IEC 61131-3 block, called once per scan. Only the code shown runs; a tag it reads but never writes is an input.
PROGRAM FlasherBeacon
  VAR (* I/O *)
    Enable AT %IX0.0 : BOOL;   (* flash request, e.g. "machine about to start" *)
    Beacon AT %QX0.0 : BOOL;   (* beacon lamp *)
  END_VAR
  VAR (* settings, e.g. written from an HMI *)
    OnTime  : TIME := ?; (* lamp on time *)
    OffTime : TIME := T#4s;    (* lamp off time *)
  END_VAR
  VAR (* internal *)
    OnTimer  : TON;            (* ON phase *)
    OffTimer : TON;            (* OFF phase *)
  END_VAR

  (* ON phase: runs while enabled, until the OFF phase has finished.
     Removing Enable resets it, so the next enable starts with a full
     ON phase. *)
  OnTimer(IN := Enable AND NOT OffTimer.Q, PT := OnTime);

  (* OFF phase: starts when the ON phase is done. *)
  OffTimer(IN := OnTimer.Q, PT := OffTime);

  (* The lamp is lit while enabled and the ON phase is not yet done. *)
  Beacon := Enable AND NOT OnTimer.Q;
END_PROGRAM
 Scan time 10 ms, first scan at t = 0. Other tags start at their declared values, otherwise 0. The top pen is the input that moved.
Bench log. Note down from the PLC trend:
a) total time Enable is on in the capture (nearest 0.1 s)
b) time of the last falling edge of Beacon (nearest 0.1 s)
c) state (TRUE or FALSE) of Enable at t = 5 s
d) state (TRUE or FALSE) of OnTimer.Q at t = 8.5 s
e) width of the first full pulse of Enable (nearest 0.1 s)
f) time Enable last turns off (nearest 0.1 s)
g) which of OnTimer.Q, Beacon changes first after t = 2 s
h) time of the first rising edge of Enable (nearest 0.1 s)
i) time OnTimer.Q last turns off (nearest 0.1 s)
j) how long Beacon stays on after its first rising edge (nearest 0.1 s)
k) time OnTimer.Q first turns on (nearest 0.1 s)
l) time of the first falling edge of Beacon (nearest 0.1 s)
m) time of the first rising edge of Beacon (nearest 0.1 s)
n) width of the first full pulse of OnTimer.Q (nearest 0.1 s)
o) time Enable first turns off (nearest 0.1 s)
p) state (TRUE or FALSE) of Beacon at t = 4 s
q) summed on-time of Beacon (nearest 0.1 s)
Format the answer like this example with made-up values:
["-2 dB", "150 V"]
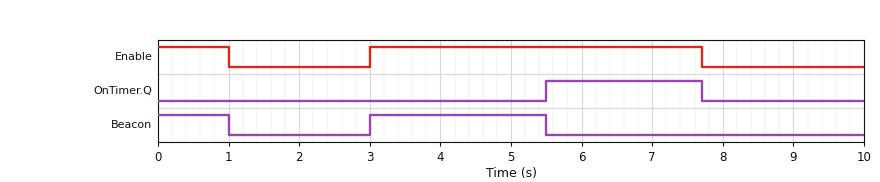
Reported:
["5.7 s", "5.5 s", "TRUE", "FALSE", "4.7 s", "7.7 s", "Beacon", "3.0 s", "7.7 s", "2.5 s", "5.5 s", "1.0 s", "3.0 s", "2.2 s", "1.0 s", "TRUE", "3.5 s"]
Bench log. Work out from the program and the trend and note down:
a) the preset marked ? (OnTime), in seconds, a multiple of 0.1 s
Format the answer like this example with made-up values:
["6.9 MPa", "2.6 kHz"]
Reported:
["2.5 s"]
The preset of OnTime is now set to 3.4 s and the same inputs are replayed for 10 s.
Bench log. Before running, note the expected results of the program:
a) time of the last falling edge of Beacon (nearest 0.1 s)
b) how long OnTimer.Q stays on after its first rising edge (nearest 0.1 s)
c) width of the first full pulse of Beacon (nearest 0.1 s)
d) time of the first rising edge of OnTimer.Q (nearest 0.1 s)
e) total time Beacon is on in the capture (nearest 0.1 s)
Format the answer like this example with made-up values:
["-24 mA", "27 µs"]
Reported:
["6.4 s", "1.3 s", "3.4 s", "6.4 s", "4.4 s"]
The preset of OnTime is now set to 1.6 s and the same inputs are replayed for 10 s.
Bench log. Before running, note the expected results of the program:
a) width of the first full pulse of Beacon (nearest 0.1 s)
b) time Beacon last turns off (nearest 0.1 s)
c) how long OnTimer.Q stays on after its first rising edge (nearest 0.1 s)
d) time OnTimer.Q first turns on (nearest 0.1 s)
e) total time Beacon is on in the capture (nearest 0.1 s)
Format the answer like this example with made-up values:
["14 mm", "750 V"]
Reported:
["1.6 s", "4.6 s", "3.1 s", "4.6 s", "2.6 s"]
